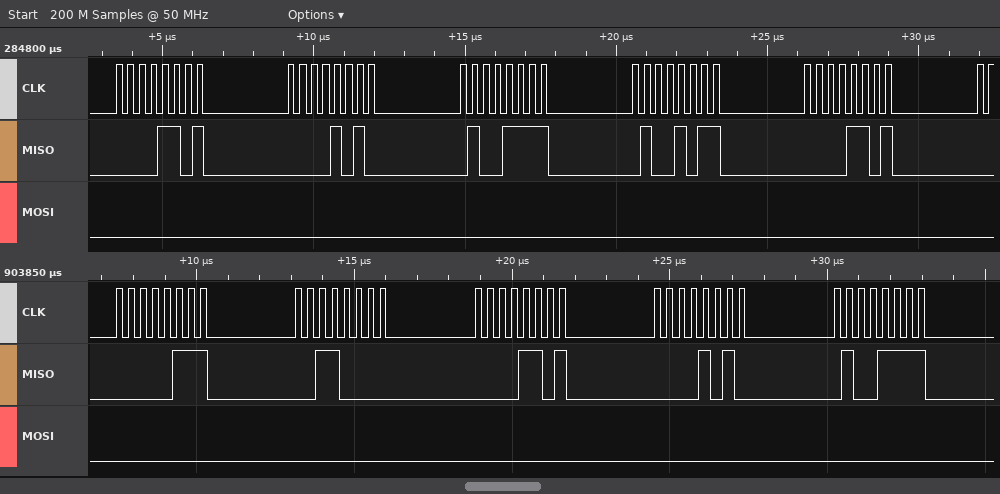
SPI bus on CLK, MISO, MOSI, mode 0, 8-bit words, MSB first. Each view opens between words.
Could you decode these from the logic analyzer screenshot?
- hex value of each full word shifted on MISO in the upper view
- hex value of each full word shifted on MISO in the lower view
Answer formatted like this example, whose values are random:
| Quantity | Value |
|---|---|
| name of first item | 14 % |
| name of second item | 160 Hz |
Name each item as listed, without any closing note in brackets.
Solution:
| Quantity | Value |
|---|---|
| hex value of each full word shifted on MISO in the upper view | 0D, 0A, 4F, 4B, 0D |
| hex value of each full word shifted on MISO in the lower view | 07, 30, 0D, 0A, 4F |
